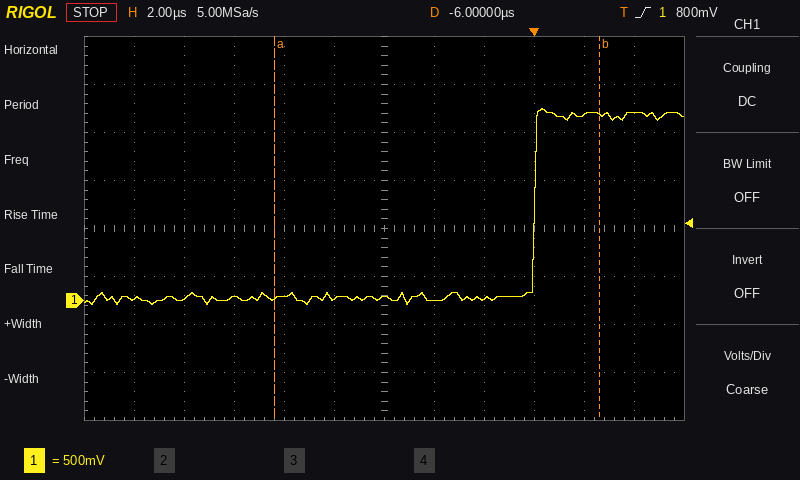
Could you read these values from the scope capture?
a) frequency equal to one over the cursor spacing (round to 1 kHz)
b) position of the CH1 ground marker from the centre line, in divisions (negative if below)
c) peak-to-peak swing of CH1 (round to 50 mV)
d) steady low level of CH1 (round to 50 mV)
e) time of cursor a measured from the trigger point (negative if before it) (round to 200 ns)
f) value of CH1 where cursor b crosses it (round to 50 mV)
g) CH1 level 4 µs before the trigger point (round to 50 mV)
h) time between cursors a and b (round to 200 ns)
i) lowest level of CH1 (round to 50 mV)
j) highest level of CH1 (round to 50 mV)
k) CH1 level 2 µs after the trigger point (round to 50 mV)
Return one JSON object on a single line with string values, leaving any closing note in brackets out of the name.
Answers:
{"frequency equal to one over the cursor spacing": "77 kHz", "position of the CH1 ground marker from the centre line, in divisions": "-1.5 div", "peak-to-peak swing of CH1": "2.05 V", "steady low level of CH1": "50 mV", "time of cursor a measured from the trigger point (negative if before it)": "-10.4 µs", "value of CH1 where cursor b crosses it": "1.95 V", "CH1 level 4 µs before the trigger point": "0 mV", "time between cursors a and b": "13.0 µs", "lowest level of CH1": "-50 mV", "highest level of CH1": "2.00 V", "CH1 level 2 µs after the trigger point": "1.95 V"}
